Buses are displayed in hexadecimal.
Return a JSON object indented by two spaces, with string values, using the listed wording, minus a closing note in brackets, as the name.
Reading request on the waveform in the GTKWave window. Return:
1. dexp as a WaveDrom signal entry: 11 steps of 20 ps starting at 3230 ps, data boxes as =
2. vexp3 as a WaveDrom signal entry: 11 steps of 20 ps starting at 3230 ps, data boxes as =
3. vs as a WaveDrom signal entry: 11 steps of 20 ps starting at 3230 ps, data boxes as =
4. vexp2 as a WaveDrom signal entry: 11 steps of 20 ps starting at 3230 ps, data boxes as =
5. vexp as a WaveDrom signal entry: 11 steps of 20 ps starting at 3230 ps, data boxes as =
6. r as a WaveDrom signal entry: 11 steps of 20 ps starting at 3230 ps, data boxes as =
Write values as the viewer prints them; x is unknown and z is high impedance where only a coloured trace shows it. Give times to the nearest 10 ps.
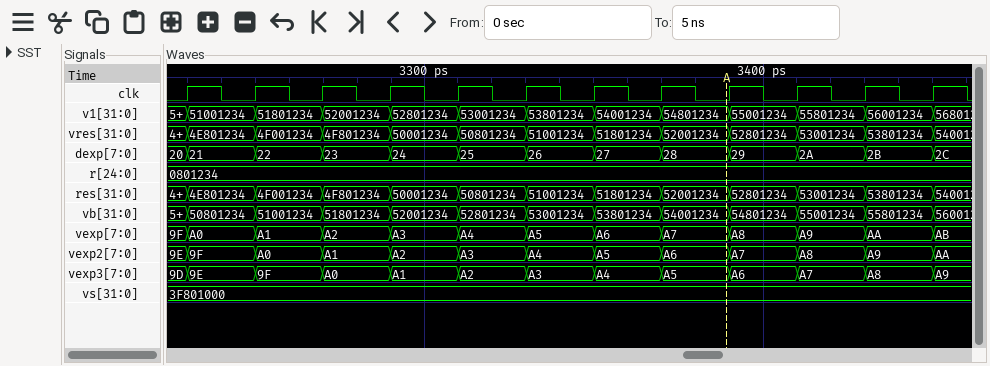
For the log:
{
  "dexp as a WaveDrom signal entry: 11 steps of 20 ps starting at 3230 ps, data boxes as =": "{name: 'dexp', wave: '===========', data: '21 22 23 24 25 26 27 28 29 2A 2B'}",
  "vexp3 as a WaveDrom signal entry: 11 steps of 20 ps starting at 3230 ps, data boxes as =": "{name: 'vexp3', wave: '===========', data: '9E 9F A0 A1 A2 A3 A4 A5 A6 A7 A8'}",
  "vs as a WaveDrom signal entry: 11 steps of 20 ps starting at 3230 ps, data boxes as =": "{name: 'vs', wave: '=..........', data: '3F801000'}",
  "vexp2 as a WaveDrom signal entry: 11 steps of 20 ps starting at 3230 ps, data boxes as =": "{name: 'vexp2', wave: '===========', data: '9F A0 A1 A2 A3 A4 A5 A6 A7 A8 A9'}",
  "vexp as a WaveDrom signal entry: 11 steps of 20 ps starting at 3230 ps, data boxes as =": "{name: 'vexp', wave: '===========', data: 'A0 A1 A2 A3 A4 A5 A6 A7 A8 A9 AA'}",
  "r as a WaveDrom signal entry: 11 steps of 20 ps starting at 3230 ps, data boxes as =": "{name: 'r', wave: '=..........', data: '0801234'}"
}
